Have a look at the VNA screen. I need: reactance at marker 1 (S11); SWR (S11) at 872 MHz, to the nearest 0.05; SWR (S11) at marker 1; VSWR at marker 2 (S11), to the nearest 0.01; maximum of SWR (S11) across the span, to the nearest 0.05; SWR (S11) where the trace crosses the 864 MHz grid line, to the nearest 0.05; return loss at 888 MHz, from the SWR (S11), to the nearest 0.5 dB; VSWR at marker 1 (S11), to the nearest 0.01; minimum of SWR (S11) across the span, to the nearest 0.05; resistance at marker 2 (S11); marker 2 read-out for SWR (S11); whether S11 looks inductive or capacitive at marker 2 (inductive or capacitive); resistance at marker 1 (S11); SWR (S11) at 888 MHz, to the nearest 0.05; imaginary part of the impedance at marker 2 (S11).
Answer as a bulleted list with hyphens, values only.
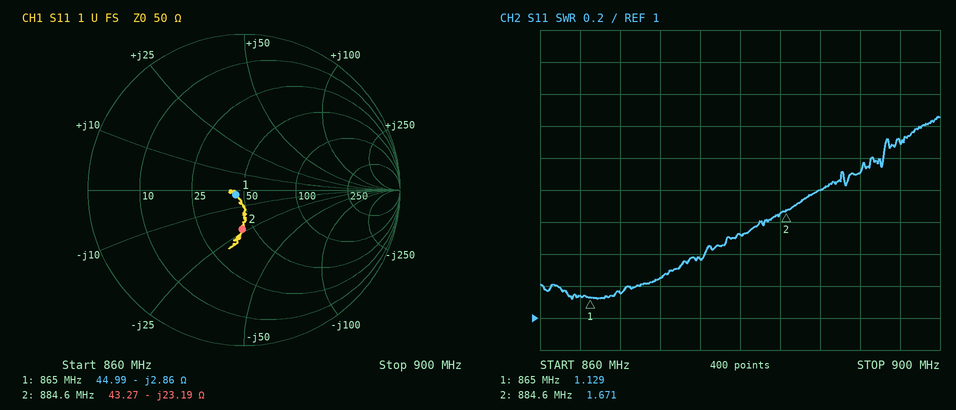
- -2.86 Ω
- 1.25
- 1.129
- 1.67
- 2.25
- 1.15
- 11.0 dB
- 1.13
- 1.10
- 43.27 Ω
- 1.671
- capacitive
- 44.99 Ω
- 1.80
- -23.19 Ω
